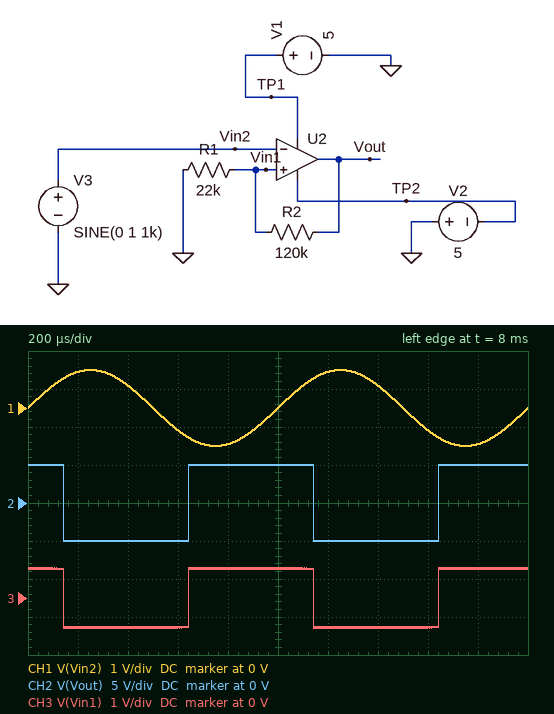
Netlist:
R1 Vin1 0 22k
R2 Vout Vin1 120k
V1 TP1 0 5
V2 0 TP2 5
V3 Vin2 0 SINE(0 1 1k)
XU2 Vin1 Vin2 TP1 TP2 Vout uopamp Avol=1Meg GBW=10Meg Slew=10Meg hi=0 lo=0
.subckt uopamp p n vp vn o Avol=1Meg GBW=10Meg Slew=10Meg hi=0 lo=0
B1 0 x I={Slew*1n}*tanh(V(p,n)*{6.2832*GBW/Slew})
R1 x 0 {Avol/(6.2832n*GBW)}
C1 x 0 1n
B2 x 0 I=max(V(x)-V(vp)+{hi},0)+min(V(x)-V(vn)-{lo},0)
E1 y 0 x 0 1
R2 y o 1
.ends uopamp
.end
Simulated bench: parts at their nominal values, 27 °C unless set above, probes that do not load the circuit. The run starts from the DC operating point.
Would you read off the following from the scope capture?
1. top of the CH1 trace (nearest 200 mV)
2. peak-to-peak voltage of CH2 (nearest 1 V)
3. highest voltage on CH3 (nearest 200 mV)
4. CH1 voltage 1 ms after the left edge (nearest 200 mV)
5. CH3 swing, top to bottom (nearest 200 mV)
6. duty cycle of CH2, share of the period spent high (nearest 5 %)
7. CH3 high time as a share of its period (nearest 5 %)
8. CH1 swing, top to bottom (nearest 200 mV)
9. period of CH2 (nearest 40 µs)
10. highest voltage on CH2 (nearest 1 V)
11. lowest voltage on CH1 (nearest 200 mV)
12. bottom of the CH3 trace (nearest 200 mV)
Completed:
1.0 V
10 V
800 mV
0 V
1.6 V
50 %
50 %
2.0 V
1.00 ms
5 V
-1.0 V
-800 mV
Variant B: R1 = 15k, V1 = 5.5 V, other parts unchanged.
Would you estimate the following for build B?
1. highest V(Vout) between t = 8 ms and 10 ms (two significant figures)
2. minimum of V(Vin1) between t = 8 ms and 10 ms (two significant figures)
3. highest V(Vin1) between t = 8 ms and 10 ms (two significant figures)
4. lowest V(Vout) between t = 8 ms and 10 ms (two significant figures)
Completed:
5.5 V
-560 mV
610 mV
-5.0 V
